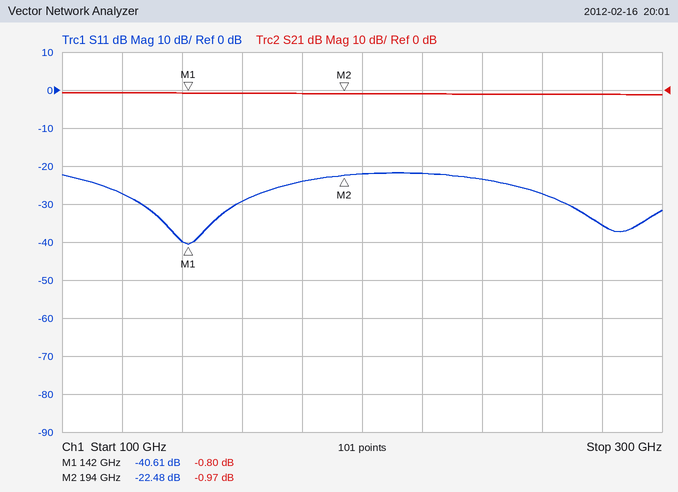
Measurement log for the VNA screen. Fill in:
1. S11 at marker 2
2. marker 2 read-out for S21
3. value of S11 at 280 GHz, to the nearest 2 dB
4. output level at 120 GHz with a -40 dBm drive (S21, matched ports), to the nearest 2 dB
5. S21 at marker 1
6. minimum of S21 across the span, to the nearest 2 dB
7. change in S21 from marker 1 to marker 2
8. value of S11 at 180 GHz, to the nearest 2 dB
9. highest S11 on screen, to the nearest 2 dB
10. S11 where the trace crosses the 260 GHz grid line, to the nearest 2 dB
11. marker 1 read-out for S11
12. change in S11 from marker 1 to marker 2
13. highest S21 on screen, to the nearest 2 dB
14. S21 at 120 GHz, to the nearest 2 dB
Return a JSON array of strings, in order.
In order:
["-22.48 dB", "-0.97 dB", "-36 dB", "-40 dBm", "-0.80 dB", "-2 dB", "-0.17 dB", "-24 dB", "-22 dB", "-28 dB", "-40.61 dB", "18.13 dB", "0 dB", "0 dB"]
